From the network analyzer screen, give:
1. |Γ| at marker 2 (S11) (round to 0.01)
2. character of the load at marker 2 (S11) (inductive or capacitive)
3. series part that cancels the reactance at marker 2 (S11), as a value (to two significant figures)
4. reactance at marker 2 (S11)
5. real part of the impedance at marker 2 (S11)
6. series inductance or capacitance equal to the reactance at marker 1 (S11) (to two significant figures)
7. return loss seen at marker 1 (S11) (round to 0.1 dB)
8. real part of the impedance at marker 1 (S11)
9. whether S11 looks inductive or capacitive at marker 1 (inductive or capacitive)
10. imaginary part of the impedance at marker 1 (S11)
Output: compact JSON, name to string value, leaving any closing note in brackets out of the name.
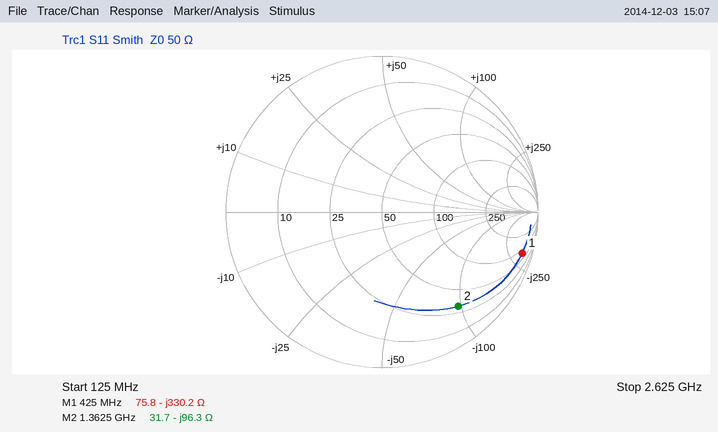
{"|Γ| at marker 2 (S11)": "0.78", "character of the load at marker 2 (S11)": "capacitive", "series part that cancels the reactance at marker 2 (S11), as a value": "11 nH", "reactance at marker 2": "-96.3 Ω", "real part of the impedance at marker 2": "31.7 Ω", "series inductance or capacitance equal to the reactance at marker 1 (S11)": "1.1 pF", "return loss seen at marker 1 (S11)": "0.6 dB", "real part of the impedance at marker 1": "75.8 Ω", "whether S11 looks inductive or capacitive at marker 1": "capacitive", "imaginary part of the impedance at marker 1": "-330.2 Ω"}
